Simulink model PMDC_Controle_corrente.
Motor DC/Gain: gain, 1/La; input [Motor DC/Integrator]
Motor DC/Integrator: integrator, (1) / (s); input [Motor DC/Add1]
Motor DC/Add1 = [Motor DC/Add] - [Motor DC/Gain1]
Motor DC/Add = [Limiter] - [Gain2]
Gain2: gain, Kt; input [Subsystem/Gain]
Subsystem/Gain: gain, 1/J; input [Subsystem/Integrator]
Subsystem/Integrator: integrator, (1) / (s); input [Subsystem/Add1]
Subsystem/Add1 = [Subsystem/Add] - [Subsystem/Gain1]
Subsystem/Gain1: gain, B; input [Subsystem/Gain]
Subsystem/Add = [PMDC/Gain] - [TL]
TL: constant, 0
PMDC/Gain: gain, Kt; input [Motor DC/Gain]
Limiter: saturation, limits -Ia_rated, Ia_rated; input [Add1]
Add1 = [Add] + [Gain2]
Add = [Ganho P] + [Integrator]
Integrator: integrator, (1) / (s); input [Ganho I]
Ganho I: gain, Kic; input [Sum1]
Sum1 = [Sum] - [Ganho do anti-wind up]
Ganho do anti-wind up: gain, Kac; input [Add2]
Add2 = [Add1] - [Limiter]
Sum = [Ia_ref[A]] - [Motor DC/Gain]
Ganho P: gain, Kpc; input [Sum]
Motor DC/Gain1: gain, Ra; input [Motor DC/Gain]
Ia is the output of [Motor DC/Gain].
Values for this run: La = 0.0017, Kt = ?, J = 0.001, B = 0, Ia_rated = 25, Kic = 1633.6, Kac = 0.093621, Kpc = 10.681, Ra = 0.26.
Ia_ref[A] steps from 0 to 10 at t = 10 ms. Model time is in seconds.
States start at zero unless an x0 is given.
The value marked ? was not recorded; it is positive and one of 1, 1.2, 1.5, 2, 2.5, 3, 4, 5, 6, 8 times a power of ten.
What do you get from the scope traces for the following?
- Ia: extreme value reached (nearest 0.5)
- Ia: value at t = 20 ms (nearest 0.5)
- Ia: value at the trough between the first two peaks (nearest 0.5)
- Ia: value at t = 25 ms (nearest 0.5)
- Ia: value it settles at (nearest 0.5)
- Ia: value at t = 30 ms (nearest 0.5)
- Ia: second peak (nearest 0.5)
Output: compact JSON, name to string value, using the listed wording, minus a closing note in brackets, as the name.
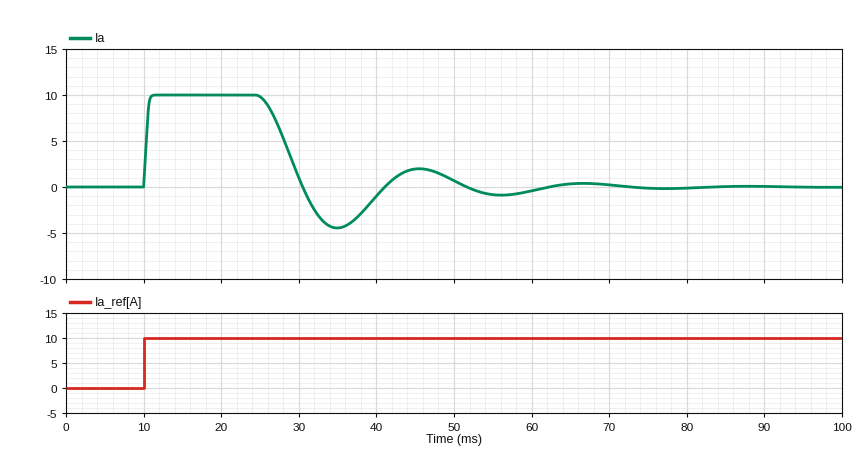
{"Ia: extreme value reached": "10.0", "Ia: value at t = 20 ms": "10.0", "Ia: value at the trough between the first two peaks": "-4.5", "Ia: value at t = 25 ms": "10.0", "Ia: value it settles at": "0.0", "Ia: value at t = 30 ms": "1.0", "Ia: second peak": "2.0"}
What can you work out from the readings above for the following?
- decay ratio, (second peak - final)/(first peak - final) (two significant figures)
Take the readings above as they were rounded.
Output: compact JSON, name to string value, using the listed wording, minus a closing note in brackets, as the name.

{"decay ratio, (second peak - final)/(first peak - final)": "0.20"}
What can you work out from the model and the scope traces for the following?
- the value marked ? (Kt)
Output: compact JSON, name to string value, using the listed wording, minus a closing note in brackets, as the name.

{"the value marked ?": "0.4"}
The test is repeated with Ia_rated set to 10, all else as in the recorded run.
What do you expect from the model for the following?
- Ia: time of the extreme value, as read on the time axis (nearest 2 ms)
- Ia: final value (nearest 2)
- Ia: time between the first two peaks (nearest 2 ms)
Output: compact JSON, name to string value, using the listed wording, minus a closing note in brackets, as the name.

{"Ia: time of the extreme value, as read on the time axis": "14 ms", "Ia: final value": "0", "Ia: time between the first two peaks": "22 ms"}
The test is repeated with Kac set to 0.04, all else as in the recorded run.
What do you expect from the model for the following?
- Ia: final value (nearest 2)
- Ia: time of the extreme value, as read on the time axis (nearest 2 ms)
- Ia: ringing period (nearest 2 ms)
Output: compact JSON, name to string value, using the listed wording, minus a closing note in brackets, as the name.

{"Ia: final value": "0", "Ia: time of the extreme value, as read on the time axis": "12 ms", "Ia: ringing period": "34 ms"}
